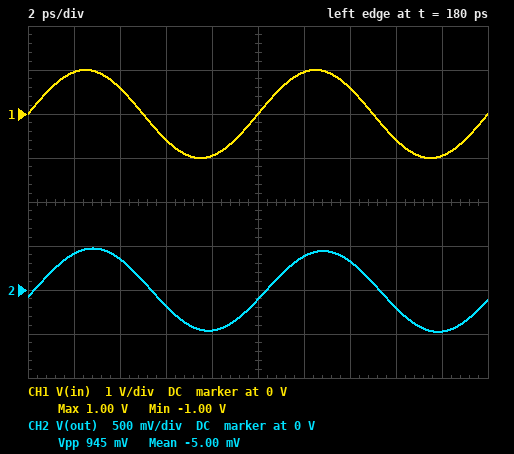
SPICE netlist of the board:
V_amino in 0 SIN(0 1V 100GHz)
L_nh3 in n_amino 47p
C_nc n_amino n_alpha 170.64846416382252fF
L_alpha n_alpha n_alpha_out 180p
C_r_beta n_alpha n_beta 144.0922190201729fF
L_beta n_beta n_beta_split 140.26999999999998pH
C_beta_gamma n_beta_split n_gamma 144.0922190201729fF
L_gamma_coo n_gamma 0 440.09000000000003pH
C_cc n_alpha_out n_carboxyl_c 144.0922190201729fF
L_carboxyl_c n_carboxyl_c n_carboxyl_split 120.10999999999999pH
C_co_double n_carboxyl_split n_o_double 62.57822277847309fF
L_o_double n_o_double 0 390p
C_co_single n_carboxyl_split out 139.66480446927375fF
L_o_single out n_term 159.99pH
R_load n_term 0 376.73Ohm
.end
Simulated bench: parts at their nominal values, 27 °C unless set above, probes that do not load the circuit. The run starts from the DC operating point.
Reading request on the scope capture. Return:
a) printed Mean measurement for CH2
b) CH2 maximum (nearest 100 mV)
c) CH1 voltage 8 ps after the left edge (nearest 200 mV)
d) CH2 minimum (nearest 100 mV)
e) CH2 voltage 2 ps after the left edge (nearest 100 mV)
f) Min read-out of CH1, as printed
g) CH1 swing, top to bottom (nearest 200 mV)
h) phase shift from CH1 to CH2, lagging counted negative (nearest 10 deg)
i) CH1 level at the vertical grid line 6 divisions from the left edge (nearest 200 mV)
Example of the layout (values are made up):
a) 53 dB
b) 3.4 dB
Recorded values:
a) -5.00 mV
b) 500 mV
c) -1.0 V
d) -500 mV
e) 400 mV
f) -1.00 V
g) 2.0 V
h) -10 deg
i) 1.0 V
